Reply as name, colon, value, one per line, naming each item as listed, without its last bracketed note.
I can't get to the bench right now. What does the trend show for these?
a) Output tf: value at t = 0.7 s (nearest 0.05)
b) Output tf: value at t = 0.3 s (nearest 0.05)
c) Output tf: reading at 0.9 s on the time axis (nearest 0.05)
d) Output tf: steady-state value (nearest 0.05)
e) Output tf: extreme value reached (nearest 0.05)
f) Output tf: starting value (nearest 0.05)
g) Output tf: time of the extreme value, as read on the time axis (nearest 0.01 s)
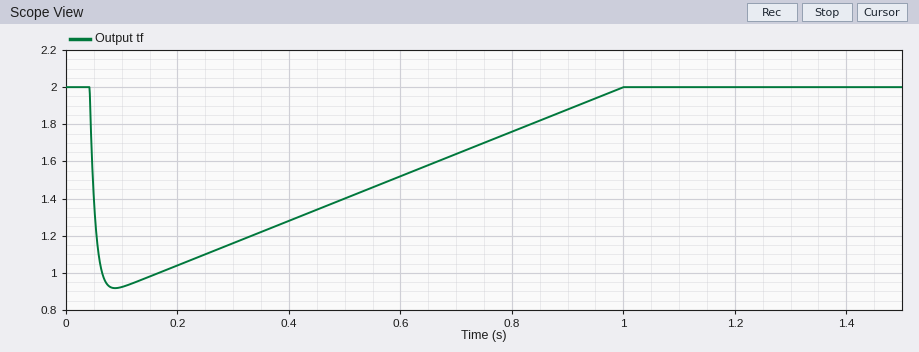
Output tf: value at t = 0.7 s: 1.65
Output tf: value at t = 0.3 s: 1.15
Output tf: reading at 0.9 s on the time axis: 1.90
Output tf: steady-state value: 2.00
Output tf: extreme value reached: 0.90
Output tf: starting value: 2.00
Output tf: time of the extreme value, as read on the time axis: 0.09 s
